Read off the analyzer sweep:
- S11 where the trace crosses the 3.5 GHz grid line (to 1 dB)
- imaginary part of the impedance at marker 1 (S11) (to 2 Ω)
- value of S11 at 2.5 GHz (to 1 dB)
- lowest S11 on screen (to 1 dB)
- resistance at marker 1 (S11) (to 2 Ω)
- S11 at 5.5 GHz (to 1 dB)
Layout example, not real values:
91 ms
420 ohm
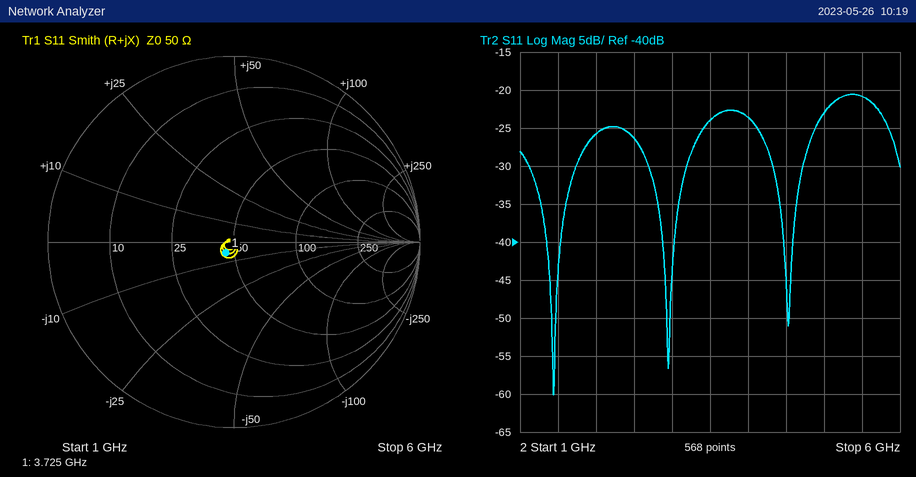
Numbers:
-24 dB
-6 Ω
-26 dB
-60 dB
46 Ω
-21 dB
